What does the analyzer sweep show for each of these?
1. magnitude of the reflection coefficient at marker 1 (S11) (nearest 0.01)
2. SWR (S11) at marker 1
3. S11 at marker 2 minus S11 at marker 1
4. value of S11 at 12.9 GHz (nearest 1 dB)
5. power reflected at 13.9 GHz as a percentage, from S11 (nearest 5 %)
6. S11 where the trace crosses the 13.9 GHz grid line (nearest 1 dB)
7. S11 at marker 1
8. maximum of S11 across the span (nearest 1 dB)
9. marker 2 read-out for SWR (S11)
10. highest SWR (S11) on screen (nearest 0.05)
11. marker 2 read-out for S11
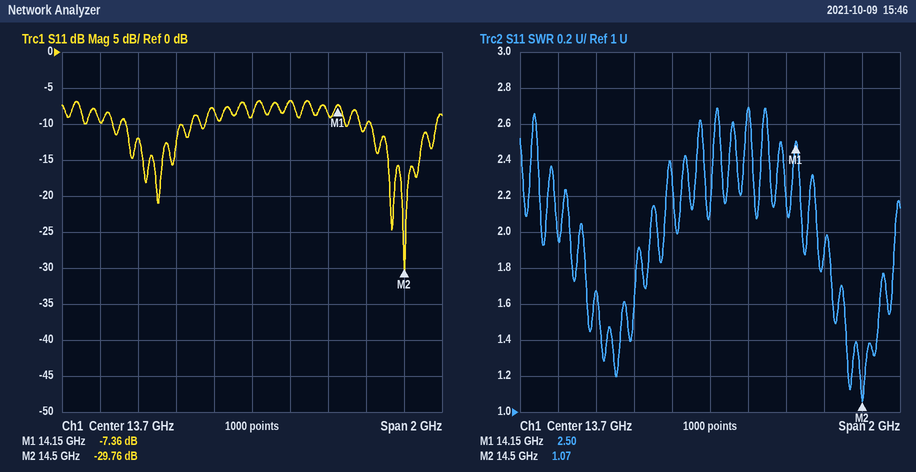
0.43
2.50
-22.40 dB
-10 dB
20 %
-7 dB
-7.36 dB
-7 dB
1.07
2.70
-29.76 dB
